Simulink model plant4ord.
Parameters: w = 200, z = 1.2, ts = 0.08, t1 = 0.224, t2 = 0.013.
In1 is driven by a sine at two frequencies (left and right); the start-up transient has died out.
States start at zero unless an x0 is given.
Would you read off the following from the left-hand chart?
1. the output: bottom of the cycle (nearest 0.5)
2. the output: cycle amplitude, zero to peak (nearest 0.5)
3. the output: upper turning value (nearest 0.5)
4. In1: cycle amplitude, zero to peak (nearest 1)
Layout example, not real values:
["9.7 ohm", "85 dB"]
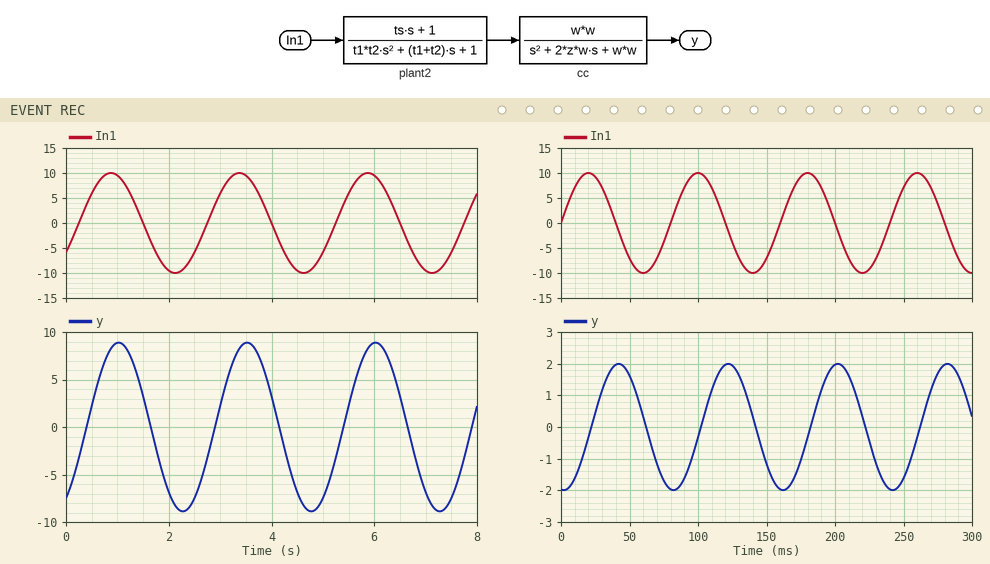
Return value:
["-9.0", "9.0", "9.0", "10"]
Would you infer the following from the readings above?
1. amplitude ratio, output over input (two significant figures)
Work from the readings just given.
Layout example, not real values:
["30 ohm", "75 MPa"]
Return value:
["0.90"]
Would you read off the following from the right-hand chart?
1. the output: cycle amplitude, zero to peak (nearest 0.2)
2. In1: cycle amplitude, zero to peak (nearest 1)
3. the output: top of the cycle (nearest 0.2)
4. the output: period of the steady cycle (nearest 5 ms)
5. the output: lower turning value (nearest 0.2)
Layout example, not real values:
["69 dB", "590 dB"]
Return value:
["2.0", "10", "2.0", "80 ms", "-2.0"]
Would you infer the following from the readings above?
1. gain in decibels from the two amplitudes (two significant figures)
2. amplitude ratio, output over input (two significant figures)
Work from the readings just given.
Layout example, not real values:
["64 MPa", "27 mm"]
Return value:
["-14 dB", "0.20"]
